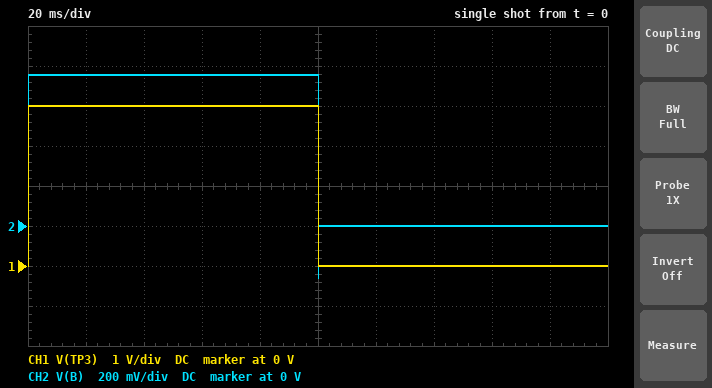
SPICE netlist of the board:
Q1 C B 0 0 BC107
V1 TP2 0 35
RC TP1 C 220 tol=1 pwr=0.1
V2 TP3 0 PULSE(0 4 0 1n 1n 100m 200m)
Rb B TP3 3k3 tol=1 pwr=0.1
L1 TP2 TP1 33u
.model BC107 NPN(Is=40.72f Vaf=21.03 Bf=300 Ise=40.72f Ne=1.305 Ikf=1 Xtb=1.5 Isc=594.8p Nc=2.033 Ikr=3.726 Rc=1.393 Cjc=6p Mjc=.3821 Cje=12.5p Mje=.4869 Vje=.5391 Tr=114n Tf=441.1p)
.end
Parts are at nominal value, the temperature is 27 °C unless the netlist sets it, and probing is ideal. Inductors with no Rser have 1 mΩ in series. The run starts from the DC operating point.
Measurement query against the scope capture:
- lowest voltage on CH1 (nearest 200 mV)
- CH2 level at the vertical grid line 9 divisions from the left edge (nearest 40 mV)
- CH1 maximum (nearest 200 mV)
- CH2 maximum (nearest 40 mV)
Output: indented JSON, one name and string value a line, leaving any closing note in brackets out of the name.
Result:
{
  "lowest voltage on CH1": "0 V",
  "CH2 level at the vertical grid line 9 divisions from the left edge": "0 V",
  "CH1 maximum": "4.0 V",
  "CH2 maximum": "760 mV"
}
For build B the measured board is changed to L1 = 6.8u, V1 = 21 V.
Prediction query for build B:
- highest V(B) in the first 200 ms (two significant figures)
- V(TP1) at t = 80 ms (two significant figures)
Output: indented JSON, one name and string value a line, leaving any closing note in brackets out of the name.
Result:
{
  "highest V(B) in the first 200 ms": "740 mV",
  "V(TP1) at t = 80 ms": "21 V"
}
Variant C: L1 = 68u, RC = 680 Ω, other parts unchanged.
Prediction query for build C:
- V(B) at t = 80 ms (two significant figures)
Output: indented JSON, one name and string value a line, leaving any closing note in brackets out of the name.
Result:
{
  "V(B) at t = 80 ms": "720 mV"
}
